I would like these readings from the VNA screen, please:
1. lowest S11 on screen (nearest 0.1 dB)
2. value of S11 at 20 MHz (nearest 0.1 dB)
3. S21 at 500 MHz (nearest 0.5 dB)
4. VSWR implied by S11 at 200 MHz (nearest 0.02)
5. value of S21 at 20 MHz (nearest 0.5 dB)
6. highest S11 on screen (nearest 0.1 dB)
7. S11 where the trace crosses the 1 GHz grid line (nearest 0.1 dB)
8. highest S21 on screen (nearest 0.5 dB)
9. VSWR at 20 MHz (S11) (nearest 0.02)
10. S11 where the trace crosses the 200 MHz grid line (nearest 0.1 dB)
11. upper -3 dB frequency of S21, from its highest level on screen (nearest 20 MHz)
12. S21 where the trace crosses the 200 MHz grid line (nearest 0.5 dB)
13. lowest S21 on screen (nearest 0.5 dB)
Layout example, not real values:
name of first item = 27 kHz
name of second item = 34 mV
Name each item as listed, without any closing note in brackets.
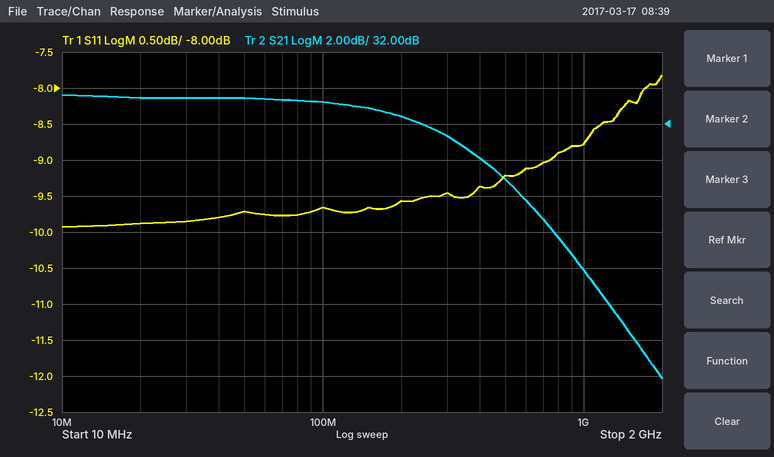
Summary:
lowest S11 on screen = -9.9 dB
value of S11 at 20 MHz = -9.9 dB
S21 at 500 MHz = 29.0 dB
VSWR implied by S11 at 200 MHz = 2.00
value of S21 at 20 MHz = 33.5 dB
highest S11 on screen = -7.8 dB
S11 where the trace crosses the 1 GHz grid line = -8.8 dB
highest S21 on screen = 33.5 dB
VSWR at 20 MHz (S11) = 1.94
S11 where the trace crosses the 200 MHz grid line = -9.6 dB
upper -3 dB frequency of S21, from its highest level on screen = 360 MHz
S21 where the trace crosses the 200 MHz grid line = 32.5 dB
lowest S21 on screen = 18.0 dB
